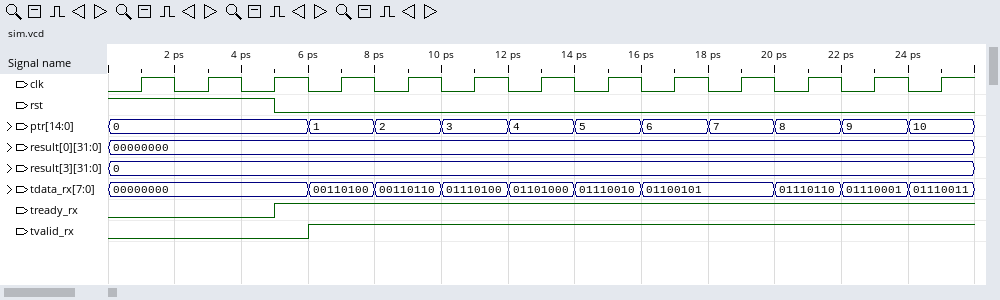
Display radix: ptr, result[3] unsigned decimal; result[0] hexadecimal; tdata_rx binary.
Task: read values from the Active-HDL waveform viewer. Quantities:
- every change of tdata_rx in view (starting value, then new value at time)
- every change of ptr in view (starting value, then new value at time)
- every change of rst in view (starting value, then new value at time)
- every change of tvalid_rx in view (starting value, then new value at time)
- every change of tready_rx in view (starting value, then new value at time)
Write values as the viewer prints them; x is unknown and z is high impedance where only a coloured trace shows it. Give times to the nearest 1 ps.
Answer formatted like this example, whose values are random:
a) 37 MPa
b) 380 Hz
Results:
a) 00000000, 00110100 at 6 ps, 00110110 at 8 ps, 01110100 at 10 ps, 01101000 at 12 ps, 01110010 at 14 ps, 01100101 at 16 ps, 01110110 at 20 ps, 01110001 at 22 ps, 01110011 at 24 ps
b) 0, 1 at 6 ps, 2 at 8 ps, 3 at 10 ps, 4 at 12 ps, 5 at 14 ps, 6 at 16 ps, 7 at 18 ps, 8 at 20 ps, 9 at 22 ps, 10 at 24 ps
c) 1, 0 at 5 ps
d) 0, 1 at 6 ps
e) 0, 1 at 5 ps
